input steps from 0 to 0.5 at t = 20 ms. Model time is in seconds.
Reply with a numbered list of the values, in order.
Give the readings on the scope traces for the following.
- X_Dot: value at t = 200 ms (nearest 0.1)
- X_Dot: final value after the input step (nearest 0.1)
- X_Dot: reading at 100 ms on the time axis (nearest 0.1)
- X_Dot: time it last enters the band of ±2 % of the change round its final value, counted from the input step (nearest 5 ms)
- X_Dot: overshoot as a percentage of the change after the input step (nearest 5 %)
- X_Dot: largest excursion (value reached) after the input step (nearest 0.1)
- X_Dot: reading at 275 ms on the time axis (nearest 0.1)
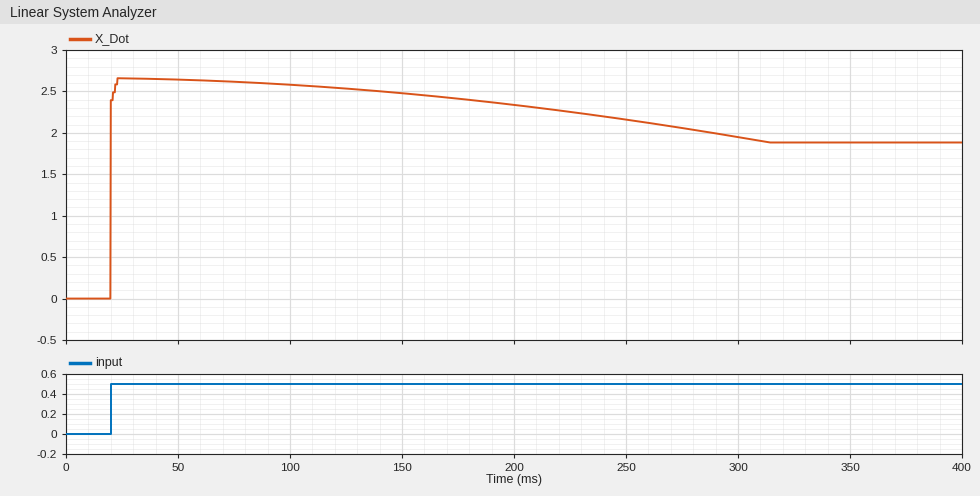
1. 2.3
2. 1.9
3. 2.6
4. 285 ms
5. 40 %
6. 2.7
7. 2.1
